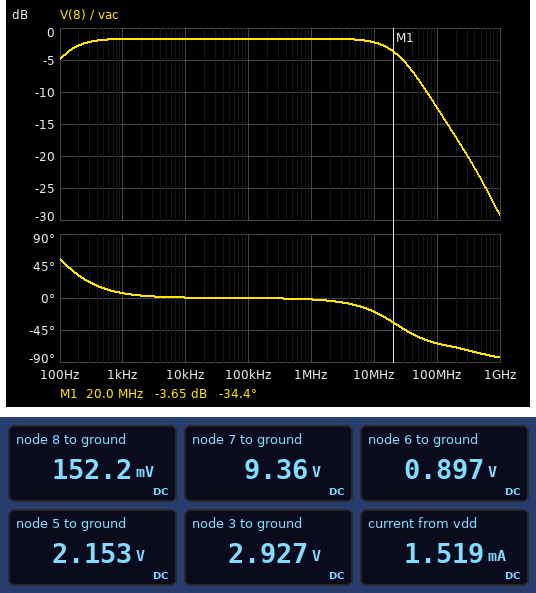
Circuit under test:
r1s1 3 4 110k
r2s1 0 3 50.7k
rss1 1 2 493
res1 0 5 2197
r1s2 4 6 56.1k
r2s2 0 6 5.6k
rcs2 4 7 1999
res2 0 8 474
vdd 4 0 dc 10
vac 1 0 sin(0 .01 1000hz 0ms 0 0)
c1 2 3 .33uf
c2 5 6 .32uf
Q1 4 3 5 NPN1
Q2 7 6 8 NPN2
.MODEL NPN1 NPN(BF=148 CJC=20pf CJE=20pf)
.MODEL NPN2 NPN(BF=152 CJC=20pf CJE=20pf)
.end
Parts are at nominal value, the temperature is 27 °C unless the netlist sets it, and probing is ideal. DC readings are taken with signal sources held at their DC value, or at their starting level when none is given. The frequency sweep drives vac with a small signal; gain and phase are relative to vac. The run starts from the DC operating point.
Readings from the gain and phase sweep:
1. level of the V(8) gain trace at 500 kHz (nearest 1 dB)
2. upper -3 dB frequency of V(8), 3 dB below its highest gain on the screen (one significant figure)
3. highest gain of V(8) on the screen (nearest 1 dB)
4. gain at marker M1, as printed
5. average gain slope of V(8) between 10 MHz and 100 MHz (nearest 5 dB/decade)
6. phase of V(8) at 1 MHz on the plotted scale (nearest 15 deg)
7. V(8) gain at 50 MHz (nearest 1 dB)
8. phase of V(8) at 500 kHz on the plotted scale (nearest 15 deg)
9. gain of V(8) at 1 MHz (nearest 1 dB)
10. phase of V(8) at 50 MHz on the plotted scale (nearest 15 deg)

-2 dB
30 MHz
-2 dB
-3.65 dB
-10 dB/decade
0 deg
-8 dB
0 deg
-2 dB
-60 deg
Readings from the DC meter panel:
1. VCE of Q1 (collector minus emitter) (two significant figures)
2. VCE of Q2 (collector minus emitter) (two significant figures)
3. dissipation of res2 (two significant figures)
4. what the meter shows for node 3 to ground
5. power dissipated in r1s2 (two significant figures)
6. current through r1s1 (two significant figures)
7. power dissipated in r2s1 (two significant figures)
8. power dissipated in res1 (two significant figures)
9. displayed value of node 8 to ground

7.8 V
9.2 V
49 µW
2.927 V
1.5 mW
64 µA
170 µW
2.1 mW
152.2 mV
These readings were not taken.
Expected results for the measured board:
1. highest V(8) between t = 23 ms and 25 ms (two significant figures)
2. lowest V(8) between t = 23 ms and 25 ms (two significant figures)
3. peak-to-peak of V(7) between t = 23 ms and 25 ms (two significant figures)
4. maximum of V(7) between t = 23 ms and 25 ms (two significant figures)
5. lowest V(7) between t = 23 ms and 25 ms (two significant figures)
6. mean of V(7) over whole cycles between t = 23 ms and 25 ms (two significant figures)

160 mV
140 mV
69 mV
9.4 V
9.3 V
9.4 V
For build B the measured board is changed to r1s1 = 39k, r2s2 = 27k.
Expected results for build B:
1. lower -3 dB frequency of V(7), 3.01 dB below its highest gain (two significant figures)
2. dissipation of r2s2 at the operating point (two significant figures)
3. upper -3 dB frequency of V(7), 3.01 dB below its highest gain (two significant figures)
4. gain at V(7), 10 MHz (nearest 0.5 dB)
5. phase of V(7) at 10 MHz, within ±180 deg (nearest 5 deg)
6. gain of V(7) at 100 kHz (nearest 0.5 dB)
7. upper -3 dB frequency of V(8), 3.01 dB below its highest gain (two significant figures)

320 Hz
270 µW
3.7 MHz
1.5 dB
45 deg
9.0 dB
27 MHz
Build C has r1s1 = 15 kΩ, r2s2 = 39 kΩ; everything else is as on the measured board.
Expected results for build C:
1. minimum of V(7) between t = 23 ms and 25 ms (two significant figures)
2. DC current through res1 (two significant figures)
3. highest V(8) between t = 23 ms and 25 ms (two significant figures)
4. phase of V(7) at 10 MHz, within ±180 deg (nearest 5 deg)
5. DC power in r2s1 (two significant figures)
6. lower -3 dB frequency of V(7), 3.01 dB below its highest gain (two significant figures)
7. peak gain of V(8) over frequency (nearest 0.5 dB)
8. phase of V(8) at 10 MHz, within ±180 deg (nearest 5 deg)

2.0 V
3.0 mA
1.9 V
40 deg
1.1 mW
3.8 MHz
-1.0 dB
-20 deg
